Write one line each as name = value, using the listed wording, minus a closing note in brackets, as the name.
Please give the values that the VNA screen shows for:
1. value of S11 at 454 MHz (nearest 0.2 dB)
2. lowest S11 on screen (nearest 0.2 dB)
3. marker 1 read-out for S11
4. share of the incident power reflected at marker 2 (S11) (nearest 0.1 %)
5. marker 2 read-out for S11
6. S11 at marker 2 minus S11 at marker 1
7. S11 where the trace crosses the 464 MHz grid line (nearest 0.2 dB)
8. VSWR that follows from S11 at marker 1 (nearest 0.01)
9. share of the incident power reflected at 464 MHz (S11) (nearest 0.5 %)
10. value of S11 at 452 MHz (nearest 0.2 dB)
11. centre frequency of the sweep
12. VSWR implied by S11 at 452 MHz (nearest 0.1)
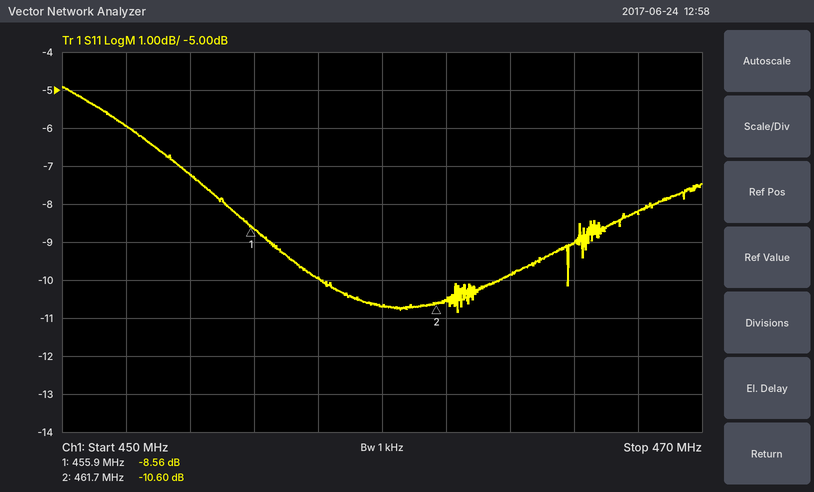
value of S11 at 454 MHz = -7.2 dB
lowest S11 on screen = -10.8 dB
marker 1 read-out for S11 = -8.56 dB
share of the incident power reflected at marker 2 (S11) = 8.7 %
marker 2 read-out for S11 = -10.60 dB
S11 at marker 2 minus S11 at marker 1 = -2.04 dB
S11 where the trace crosses the 464 MHz grid line = -9.8 dB
VSWR that follows from S11 at marker 1 = 2.19
share of the incident power reflected at 464 MHz (S11) = 10.5 %
value of S11 at 452 MHz = -6.0 dB
centre frequency of the sweep = 460 MHz
VSWR implied by S11 at 452 MHz = 3.0
